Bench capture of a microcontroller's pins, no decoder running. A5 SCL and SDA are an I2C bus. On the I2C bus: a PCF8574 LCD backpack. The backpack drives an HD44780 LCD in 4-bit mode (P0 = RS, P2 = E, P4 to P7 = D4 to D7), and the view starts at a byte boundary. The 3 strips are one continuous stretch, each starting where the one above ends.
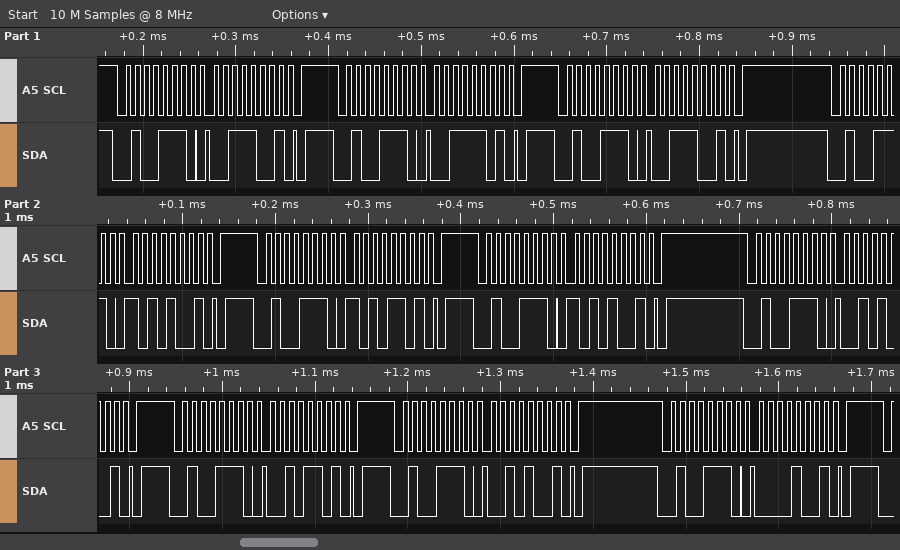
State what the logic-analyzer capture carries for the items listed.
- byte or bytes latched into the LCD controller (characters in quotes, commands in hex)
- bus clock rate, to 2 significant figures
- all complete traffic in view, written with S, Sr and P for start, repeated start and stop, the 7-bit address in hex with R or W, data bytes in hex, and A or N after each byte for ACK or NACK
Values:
':'
100 kHz
S 27W A 39 A P S 27W A 3D A P S 27W A 39 A P S 27W A A9 A P S 27W A AD A P S 27W A A9 A P S 27W A 29 A P S 27W A 2D A P S 27W A 29 A P S 27W A 09 A P
